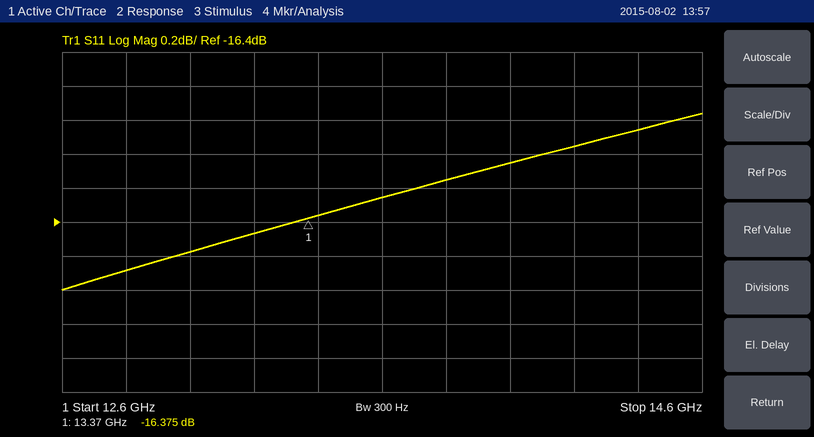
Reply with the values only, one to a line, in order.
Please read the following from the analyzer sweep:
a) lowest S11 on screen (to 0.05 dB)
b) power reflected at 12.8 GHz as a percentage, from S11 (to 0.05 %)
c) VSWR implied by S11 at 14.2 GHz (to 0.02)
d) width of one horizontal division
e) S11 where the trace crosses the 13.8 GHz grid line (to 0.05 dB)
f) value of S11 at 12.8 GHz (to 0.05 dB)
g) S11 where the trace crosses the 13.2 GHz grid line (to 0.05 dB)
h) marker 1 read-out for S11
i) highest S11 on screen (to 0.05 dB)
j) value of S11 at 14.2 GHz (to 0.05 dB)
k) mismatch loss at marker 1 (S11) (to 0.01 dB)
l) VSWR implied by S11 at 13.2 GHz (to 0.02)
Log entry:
-16.80 dB
2.15 %
1.38
200 MHz
-16.15 dB
-16.70 dB
-16.45 dB
-16.375 dB
-15.75 dB
-15.95 dB
0.10 dB
1.36
